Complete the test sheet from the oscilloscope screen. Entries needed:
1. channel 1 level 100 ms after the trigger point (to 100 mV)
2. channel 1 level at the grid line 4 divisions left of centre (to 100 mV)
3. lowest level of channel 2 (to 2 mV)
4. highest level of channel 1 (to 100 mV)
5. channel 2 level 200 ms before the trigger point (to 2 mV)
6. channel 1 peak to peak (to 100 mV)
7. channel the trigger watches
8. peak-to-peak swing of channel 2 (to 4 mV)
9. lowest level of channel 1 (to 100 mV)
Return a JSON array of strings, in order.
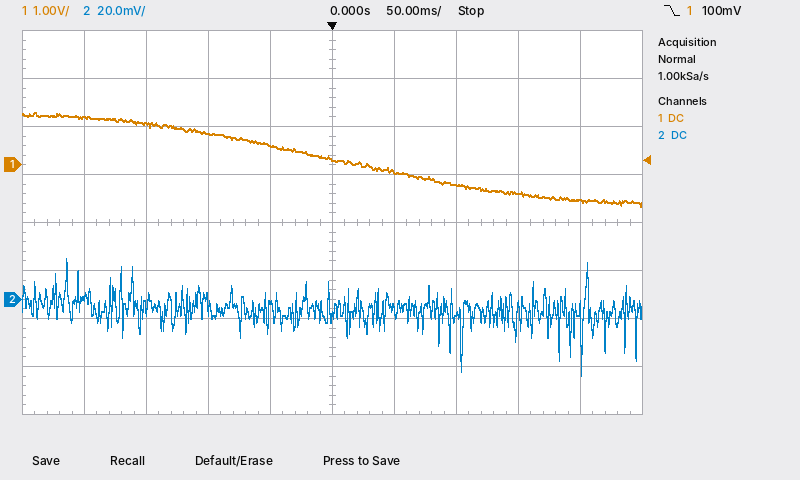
["-400 mV", "1.0 V", "-32 mV", "1.1 V", "2 mV", "2.0 V", "channel 1", "48 mV", "-900 mV"]
